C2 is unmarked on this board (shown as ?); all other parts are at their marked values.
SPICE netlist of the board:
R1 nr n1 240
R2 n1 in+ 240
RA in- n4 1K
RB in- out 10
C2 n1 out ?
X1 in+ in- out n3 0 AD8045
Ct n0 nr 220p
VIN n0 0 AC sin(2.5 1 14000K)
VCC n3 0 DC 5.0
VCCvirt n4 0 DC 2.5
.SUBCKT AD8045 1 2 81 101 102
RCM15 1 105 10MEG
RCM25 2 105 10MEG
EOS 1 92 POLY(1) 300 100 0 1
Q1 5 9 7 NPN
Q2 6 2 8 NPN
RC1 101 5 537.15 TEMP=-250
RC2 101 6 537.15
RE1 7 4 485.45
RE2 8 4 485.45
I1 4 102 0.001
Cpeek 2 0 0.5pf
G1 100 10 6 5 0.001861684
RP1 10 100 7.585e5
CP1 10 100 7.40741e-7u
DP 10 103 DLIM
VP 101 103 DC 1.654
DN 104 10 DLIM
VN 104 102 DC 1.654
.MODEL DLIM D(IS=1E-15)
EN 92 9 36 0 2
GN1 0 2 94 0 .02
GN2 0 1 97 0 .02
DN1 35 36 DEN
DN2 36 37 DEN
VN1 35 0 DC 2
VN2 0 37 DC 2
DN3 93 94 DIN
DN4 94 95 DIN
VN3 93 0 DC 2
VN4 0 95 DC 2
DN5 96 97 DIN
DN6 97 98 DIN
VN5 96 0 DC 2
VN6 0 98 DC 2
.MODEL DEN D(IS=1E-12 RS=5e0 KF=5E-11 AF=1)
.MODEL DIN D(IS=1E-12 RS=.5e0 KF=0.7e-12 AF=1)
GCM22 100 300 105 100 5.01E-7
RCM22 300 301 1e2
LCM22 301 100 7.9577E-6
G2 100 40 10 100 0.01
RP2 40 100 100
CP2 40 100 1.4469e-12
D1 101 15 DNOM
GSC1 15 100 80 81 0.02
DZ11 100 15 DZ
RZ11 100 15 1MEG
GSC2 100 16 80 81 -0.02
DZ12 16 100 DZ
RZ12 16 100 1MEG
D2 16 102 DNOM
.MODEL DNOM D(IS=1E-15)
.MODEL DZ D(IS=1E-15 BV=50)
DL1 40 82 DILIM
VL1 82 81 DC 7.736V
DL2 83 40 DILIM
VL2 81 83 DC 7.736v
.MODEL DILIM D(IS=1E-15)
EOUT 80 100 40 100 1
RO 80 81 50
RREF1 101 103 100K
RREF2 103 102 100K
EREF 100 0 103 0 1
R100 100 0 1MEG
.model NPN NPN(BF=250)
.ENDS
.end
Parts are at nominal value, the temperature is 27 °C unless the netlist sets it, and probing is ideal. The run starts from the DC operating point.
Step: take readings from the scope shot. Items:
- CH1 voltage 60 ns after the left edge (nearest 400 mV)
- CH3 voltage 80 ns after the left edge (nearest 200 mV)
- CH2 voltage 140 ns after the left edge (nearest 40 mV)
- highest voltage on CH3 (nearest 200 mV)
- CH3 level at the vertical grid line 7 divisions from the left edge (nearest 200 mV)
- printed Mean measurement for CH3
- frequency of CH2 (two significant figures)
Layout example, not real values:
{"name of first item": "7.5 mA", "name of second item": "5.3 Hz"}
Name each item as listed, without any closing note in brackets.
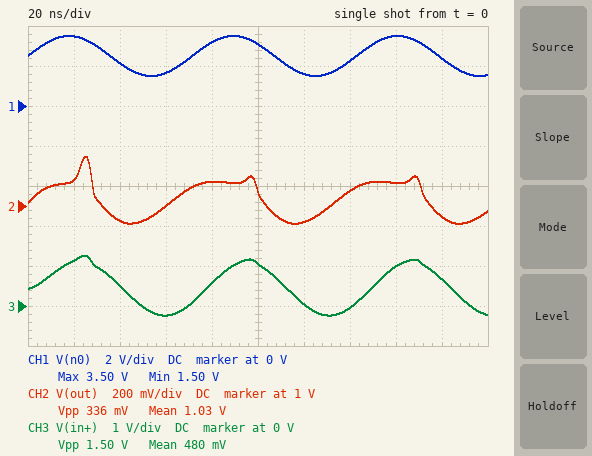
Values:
{"CH1 voltage 60 ns after the left edge": "1.6 V", "CH3 voltage 80 ns after the left edge": "600 mV", "CH2 voltage 140 ns after the left edge": "1.08 V", "highest voltage on CH3": "1.2 V", "CH3 level at the vertical grid line 7 divisions from the left edge": "0 V", "printed Mean measurement for CH3": "480 mV", "frequency of CH2": "14 MHz"}
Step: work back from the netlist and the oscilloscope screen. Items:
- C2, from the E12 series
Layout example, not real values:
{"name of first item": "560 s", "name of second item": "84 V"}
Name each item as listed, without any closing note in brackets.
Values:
{"C2, from the E12 series": "39 pF"}
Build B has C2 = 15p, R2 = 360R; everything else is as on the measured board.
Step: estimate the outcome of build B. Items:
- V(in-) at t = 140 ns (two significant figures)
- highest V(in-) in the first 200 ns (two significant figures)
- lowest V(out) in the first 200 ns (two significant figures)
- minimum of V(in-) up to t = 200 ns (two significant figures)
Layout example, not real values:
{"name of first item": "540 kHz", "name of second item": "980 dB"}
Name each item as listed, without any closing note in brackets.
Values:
{"V(in-) at t = 140 ns": "1.1 V", "highest V(in-) in the first 200 ns": "1.5 V", "lowest V(out) in the first 200 ns": "960 mV", "minimum of V(in-) up to t = 200 ns": "980 mV"}
